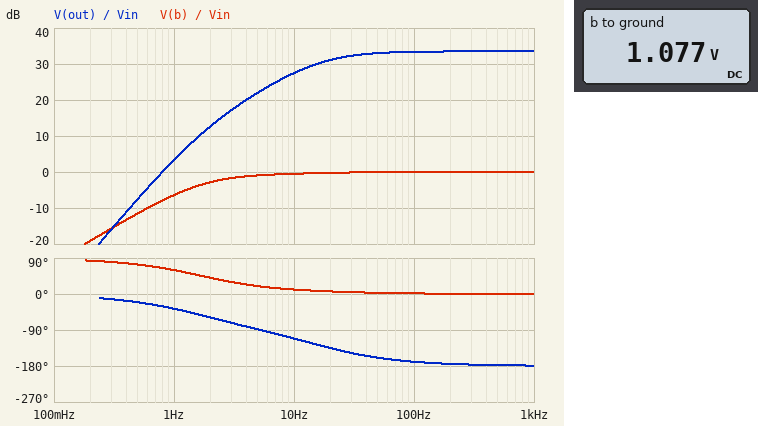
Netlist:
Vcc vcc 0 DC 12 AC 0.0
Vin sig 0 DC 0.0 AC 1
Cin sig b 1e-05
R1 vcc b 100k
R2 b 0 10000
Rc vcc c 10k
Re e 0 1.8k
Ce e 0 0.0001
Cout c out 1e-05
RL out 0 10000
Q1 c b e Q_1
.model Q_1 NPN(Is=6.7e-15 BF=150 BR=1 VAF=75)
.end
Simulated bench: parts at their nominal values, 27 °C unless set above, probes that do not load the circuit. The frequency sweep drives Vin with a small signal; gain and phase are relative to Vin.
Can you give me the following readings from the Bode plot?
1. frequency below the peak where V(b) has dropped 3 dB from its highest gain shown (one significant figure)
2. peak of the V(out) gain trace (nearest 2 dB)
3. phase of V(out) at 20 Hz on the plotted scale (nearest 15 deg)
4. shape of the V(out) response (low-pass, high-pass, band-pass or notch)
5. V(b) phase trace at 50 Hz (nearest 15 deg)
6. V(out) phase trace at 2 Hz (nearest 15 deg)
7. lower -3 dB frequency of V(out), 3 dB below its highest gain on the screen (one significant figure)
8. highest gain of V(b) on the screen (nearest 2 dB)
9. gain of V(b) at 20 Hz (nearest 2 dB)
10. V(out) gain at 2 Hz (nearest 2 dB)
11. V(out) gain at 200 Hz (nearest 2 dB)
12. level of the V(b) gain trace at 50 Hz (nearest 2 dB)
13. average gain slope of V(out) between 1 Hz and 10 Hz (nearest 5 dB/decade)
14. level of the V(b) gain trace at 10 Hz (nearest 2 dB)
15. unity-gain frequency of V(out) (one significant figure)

2 Hz
34 dB
-135 deg
high-pass
0 deg
-60 deg
20 Hz
0 dB
0 dB
12 dB
34 dB
0 dB
25 dB/decade
0 dB
800 mHz
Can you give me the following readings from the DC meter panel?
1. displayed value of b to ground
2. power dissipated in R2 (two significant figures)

1.077 V
120 µW
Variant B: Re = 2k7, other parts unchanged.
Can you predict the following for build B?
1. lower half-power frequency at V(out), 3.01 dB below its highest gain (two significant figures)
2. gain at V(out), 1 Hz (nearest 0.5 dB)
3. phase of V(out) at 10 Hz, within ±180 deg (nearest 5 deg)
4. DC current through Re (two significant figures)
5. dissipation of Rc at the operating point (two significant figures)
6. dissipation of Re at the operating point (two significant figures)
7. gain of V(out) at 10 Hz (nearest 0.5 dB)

12 Hz
2.0 dB
-120 deg
170 µA
290 µW
80 µW
26.5 dB
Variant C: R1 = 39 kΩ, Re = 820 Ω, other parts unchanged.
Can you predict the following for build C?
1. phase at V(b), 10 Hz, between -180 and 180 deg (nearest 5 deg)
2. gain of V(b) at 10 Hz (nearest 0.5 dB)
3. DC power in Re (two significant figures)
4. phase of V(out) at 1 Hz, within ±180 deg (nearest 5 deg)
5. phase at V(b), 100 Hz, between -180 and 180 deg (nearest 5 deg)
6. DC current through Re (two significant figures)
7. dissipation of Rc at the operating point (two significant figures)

25 deg
-20.0 dB
1.2 mW
110 deg
55 deg
1.2 mA
12 mW
